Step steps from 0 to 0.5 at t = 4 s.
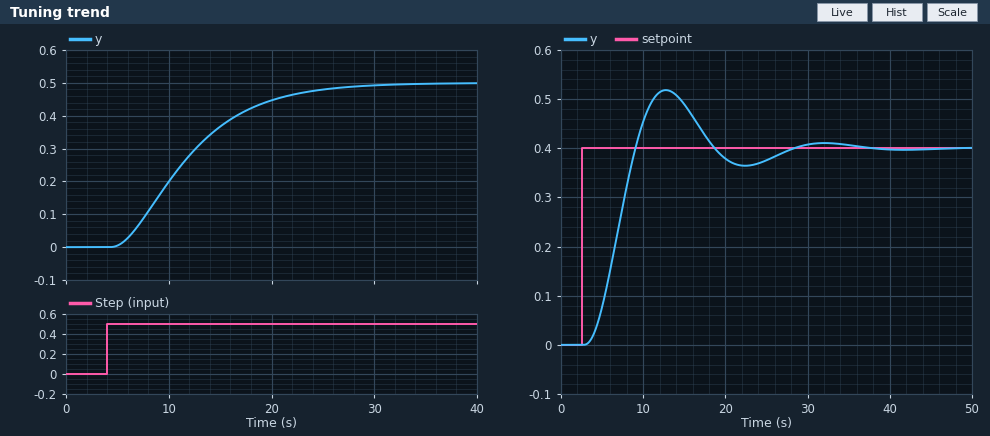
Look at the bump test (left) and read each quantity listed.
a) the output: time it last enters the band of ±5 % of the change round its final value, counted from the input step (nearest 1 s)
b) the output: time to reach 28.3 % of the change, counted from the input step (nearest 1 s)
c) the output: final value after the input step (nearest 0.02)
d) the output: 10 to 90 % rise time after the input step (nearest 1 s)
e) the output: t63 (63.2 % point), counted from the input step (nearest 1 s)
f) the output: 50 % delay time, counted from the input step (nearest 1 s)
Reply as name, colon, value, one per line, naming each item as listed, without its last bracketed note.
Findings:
the output: time it last enters the band of ±5 % of the change round its final value, counted from the input step: 20 s
the output: time to reach 28.3 % of the change, counted from the input step: 5 s
the output: final value after the input step: 0.50
the output: 10 to 90 % rise time after the input step: 14 s
the output: t63 (63.2 % point), counted from the input step: 9 s
the output: 50 % delay time, counted from the input step: 7 s
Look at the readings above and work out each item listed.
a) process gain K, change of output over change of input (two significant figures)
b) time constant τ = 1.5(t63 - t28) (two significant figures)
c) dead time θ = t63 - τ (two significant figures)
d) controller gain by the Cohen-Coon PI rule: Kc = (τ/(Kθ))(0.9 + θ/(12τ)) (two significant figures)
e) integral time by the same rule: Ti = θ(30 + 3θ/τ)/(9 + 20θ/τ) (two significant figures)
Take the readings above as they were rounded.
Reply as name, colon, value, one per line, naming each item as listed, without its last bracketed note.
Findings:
process gain K, change of output over change of input: 1.0
time constant τ = 1.5(t63 - t28): 6.0 s
dead time θ = t63 - τ: 3.0 s
controller gain by the Cohen-Coon PI rule: Kc = (τ/(Kθ))(0.9 + θ/(12τ)): 1.9
integral time by the same rule: Ti = θ(30 + 3θ/τ)/(9 + 20θ/τ): 5.0 s
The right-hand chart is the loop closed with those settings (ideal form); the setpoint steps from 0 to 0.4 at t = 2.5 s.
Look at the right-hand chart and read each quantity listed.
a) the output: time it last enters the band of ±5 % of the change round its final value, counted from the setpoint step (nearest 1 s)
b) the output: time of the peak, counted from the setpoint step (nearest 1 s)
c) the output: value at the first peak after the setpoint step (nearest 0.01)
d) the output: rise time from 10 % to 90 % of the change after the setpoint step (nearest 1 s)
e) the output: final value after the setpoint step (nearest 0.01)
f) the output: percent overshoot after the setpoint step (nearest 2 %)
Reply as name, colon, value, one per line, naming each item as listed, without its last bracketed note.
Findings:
the output: time it last enters the band of ±5 % of the change round its final value, counted from the setpoint step: 23 s
the output: time of the peak, counted from the setpoint step: 10 s
the output: value at the first peak after the setpoint step: 0.52
the output: rise time from 10 % to 90 % of the change after the setpoint step: 4 s
the output: final value after the setpoint step: 0.40
the output: percent overshoot after the setpoint step: 30 %
